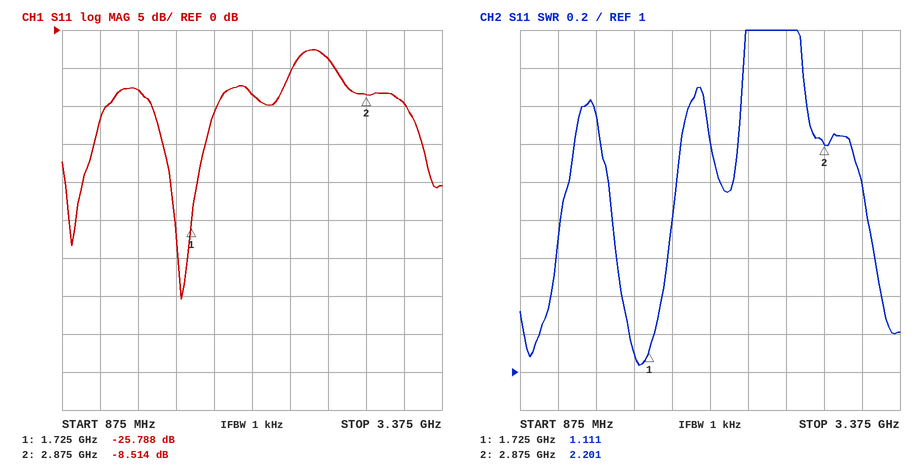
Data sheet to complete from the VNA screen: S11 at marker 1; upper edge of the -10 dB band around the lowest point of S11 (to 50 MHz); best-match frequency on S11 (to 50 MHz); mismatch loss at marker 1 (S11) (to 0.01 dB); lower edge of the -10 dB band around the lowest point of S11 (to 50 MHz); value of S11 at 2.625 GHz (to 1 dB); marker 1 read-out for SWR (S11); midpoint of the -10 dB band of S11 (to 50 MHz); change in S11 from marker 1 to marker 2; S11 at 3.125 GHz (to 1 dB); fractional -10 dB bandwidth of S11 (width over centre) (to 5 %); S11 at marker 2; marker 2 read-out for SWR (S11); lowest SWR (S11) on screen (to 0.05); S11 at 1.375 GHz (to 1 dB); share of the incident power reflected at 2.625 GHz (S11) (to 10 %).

-25.788 dB
1.90 GHz
1.65 GHz
0.01 dB
1.45 GHz
-4 dB
1.111
1.70 GHz
17.274 dB
-10 dB
25 %
-8.514 dB
2.201
1.05
-8 dB
40 %
